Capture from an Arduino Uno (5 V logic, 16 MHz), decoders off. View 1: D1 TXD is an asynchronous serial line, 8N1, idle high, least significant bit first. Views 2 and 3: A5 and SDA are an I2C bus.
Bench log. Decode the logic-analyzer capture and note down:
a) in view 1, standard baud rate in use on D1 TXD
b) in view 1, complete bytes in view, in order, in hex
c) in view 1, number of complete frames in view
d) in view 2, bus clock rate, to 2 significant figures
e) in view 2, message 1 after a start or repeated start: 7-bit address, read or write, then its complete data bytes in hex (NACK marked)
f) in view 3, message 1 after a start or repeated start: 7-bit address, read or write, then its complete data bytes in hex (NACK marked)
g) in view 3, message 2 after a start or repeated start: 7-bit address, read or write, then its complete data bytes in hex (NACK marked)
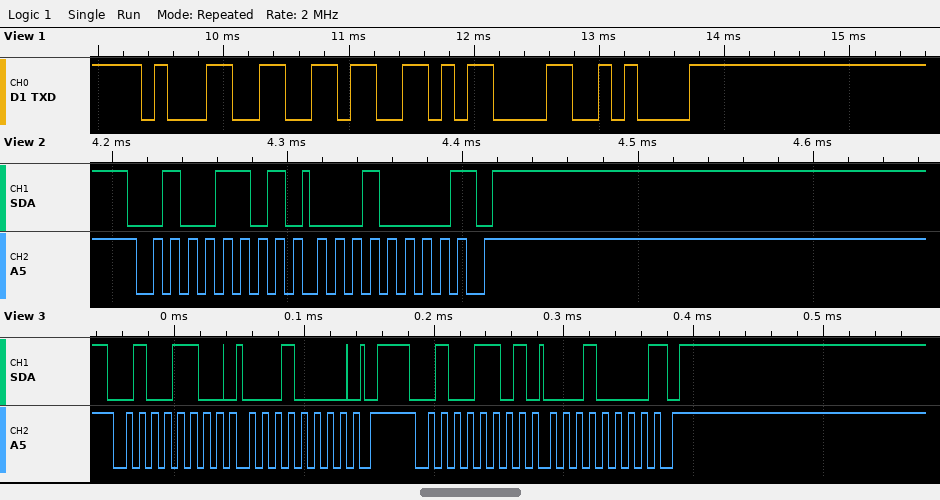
9600 baud
0x31 0x36 0x0D 0x0A
4
100 kHz
0x26 read: 10 NACK
0x26 write: 10
0x26 read: 10 NACK
